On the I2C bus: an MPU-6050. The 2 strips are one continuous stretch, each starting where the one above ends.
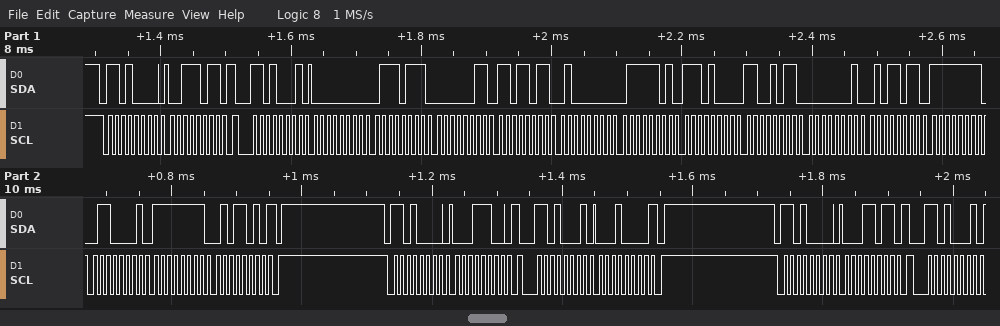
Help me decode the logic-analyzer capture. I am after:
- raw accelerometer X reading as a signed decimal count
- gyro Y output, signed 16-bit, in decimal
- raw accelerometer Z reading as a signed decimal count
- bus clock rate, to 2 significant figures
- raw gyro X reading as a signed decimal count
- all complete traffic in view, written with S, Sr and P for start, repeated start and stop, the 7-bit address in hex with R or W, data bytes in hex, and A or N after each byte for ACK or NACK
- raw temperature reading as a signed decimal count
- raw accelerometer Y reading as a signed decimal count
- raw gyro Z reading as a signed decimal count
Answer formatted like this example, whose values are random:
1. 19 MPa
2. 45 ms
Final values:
1. 119
2. -159
3. 16509
4. 100 kHz
5. 347
6. S 68W A 3B A Sr 68R A 00 A 77 A 03 A DB A 40 A 7D A E8 A CB A 01 A 5B A FF A 61 A FF A 5A N P S 68W A 1C A Sr 68R A 10 N P S 68W A 1B A Sr 68R A
7. -5941
8. 987
9. -166
